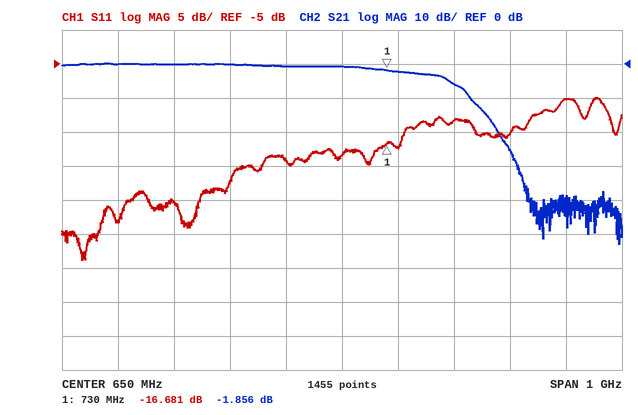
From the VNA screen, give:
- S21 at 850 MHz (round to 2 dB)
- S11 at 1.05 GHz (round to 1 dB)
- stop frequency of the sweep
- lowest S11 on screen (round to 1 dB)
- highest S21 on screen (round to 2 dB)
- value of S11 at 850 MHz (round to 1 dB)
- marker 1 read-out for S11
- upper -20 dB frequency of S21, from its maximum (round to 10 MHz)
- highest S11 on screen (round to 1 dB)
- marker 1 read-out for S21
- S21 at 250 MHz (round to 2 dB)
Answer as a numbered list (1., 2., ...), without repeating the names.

1. -6 dB
2. -10 dB
3. 1.15 GHz
4. -34 dB
5. 0 dB
6. -13 dB
7. -16.681 dB
8. 930 MHz
9. -10 dB
10. -1.856 dB
11. 0 dB
